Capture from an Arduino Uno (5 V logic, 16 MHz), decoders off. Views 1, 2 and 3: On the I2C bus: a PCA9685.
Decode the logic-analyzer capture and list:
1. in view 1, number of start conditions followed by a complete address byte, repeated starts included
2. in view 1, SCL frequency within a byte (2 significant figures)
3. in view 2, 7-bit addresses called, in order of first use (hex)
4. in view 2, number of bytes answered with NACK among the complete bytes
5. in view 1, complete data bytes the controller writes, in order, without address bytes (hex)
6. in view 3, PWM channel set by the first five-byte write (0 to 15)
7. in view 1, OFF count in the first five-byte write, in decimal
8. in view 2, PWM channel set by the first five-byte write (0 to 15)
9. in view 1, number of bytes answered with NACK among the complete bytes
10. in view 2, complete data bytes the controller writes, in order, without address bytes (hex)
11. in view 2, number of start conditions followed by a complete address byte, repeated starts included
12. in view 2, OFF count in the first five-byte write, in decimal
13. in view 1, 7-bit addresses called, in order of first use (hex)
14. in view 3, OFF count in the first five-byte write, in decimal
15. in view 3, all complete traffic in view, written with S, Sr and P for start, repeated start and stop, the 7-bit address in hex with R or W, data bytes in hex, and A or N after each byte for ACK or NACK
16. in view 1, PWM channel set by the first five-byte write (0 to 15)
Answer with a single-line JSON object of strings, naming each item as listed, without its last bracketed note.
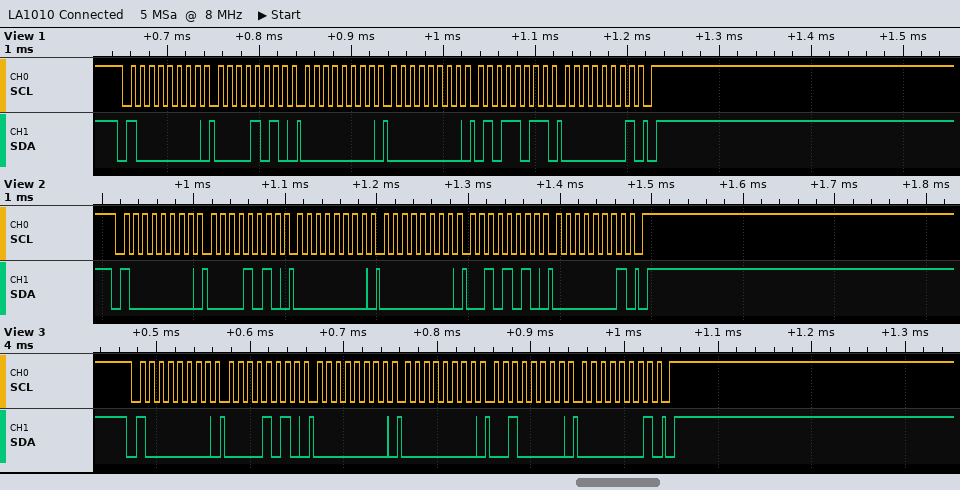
{"in view 1, number of start conditions followed by a complete address byte, repeated starts included": "1", "in view 1, SCL frequency within a byte": "100 kHz", "in view 2, 7-bit addresses called, in order of first use": "0x40", "in view 2, number of bytes answered with NACK among the complete bytes": "0", "in view 1, complete data bytes the controller writes, in order, without address bytes": "0A 00 00 5B 01", "in view 3, PWM channel set by the first five-byte write": "1", "in view 1, OFF count in the first five-byte write, in decimal": "347", "in view 2, PWM channel set by the first five-byte write": "1", "in view 1, number of bytes answered with NACK among the complete bytes": "0", "in view 2, complete data bytes the controller writes, in order, without address bytes": "0A 00 00 2A 01", "in view 2, number of start conditions followed by a complete address byte, repeated starts included": "1", "in view 2, OFF count in the first five-byte write, in decimal": "298", "in view 1, 7-bit addresses called, in order of first use": "0x40", "in view 3, OFF count in the first five-byte write, in decimal": "288", "in view 3, all complete traffic in view, written with S, Sr and P for start, repeated start and stop, the 7-bit address in hex with R or W, data bytes in hex, and A or N after each byte for ACK or NACK": "S 40W A 0A A 00 A 00 A 20 A 01 A P", "in view 1, PWM channel set by the first five-byte write": "1"}
